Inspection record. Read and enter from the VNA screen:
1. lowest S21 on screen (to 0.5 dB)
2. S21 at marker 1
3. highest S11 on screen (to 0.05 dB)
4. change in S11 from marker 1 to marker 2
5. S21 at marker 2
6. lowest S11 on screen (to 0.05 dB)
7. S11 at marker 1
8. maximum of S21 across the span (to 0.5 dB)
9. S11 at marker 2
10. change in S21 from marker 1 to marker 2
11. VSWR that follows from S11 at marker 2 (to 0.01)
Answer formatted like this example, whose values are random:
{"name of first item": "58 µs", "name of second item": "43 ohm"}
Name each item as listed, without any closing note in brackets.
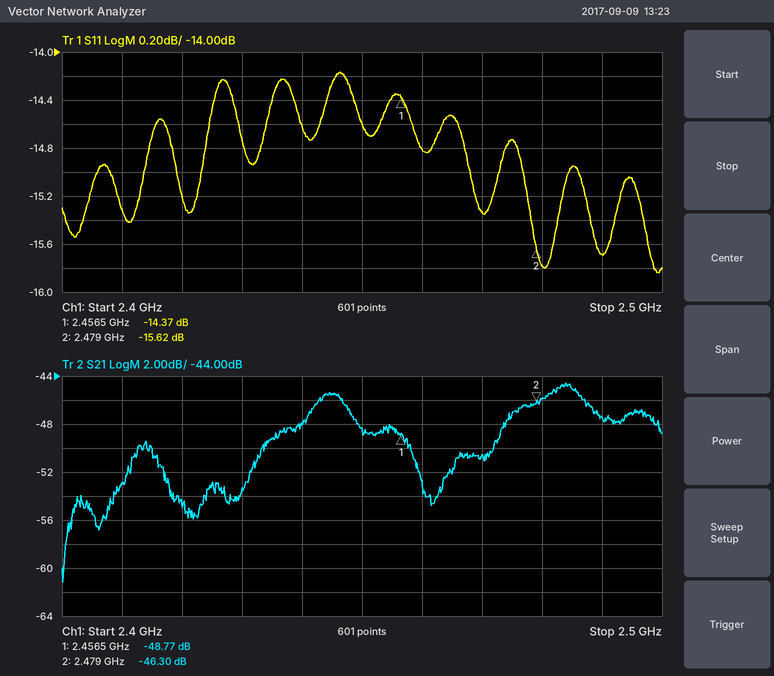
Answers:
{"lowest S21 on screen": "-61.0 dB", "S21 at marker 1": "-48.77 dB", "highest S11 on screen": "-14.15 dB", "change in S11 from marker 1 to marker 2": "-1.25 dB", "S21 at marker 2": "-46.30 dB", "lowest S11 on screen": "-15.85 dB", "S11 at marker 1": "-14.37 dB", "maximum of S21 across the span": "-44.5 dB", "S11 at marker 2": "-15.62 dB", "change in S21 from marker 1 to marker 2": "2.47 dB", "VSWR that follows from S11 at marker 2": "1.40"}
